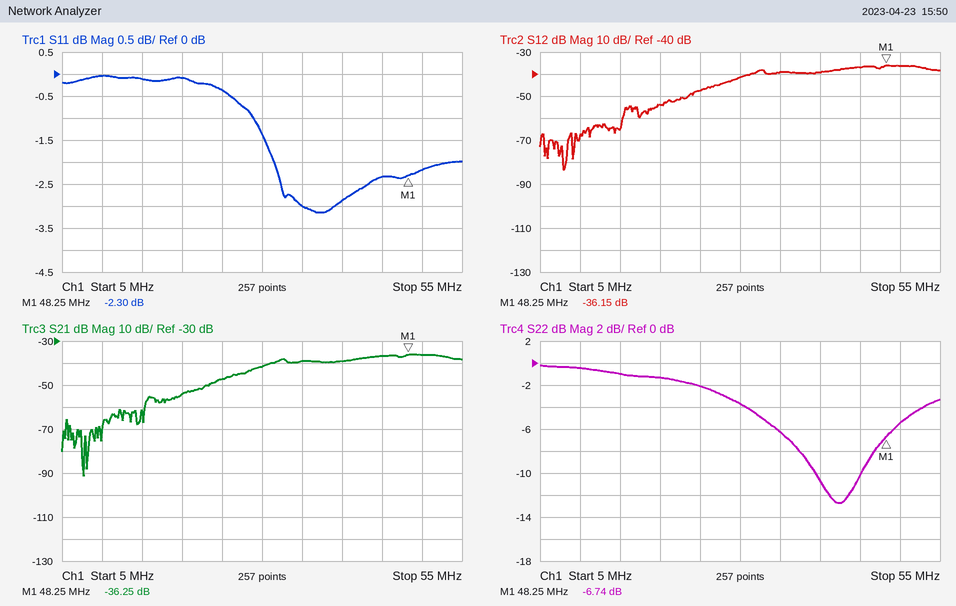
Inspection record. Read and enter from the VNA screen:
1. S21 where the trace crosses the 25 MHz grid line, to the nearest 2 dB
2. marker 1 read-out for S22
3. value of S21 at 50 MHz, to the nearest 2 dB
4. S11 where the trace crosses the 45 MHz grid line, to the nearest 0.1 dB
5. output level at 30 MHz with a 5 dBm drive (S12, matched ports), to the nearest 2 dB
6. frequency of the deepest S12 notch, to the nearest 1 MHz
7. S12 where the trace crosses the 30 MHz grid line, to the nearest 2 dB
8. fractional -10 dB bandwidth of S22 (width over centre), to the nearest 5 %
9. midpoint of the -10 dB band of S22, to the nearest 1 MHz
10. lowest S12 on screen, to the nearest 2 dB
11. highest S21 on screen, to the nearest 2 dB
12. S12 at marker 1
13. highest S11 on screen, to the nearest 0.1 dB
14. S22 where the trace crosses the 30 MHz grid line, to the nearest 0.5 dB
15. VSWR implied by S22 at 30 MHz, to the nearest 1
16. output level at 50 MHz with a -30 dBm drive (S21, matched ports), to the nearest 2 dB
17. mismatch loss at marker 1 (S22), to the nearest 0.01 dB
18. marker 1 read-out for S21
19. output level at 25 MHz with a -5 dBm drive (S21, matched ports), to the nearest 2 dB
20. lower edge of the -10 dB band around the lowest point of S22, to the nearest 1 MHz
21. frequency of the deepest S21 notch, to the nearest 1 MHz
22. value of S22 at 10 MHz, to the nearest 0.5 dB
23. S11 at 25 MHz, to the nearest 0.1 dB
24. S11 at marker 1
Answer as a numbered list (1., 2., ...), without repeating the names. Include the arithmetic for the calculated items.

1. -48 dB
2. -6.74 dB
3. -36 dB
4. -2.3 dB
5. 5 dBm + (-42 dB) = -36 dBm
6. 8 MHz
7. -42 dB
8. 6 MHz / 42 MHz ≈ 14.3 %, so 15 % to the nearest 5 %
9. 42 MHz
10. -84 dB
11. -36 dB
12. -36.15 dB
13. 0.0 dB
14. -3.5 dB
15. |Γ| = 10^(-3.5/20) = 0.6683; VSWR = (1 + 0.6683)/(1 − 0.6683) ≈ 5
16. -30 dBm + (-36 dB) = -66 dBm
17. −10 log10(1 − 10^(-6.74/10)) ≈ 1.03 dB
18. -36.25 dB
19. -5 dBm + (-48 dB) = -52 dBm
20. 39 MHz
21. 8 MHz
22. -0.5 dB
23. -0.4 dB
24. -2.30 dB
